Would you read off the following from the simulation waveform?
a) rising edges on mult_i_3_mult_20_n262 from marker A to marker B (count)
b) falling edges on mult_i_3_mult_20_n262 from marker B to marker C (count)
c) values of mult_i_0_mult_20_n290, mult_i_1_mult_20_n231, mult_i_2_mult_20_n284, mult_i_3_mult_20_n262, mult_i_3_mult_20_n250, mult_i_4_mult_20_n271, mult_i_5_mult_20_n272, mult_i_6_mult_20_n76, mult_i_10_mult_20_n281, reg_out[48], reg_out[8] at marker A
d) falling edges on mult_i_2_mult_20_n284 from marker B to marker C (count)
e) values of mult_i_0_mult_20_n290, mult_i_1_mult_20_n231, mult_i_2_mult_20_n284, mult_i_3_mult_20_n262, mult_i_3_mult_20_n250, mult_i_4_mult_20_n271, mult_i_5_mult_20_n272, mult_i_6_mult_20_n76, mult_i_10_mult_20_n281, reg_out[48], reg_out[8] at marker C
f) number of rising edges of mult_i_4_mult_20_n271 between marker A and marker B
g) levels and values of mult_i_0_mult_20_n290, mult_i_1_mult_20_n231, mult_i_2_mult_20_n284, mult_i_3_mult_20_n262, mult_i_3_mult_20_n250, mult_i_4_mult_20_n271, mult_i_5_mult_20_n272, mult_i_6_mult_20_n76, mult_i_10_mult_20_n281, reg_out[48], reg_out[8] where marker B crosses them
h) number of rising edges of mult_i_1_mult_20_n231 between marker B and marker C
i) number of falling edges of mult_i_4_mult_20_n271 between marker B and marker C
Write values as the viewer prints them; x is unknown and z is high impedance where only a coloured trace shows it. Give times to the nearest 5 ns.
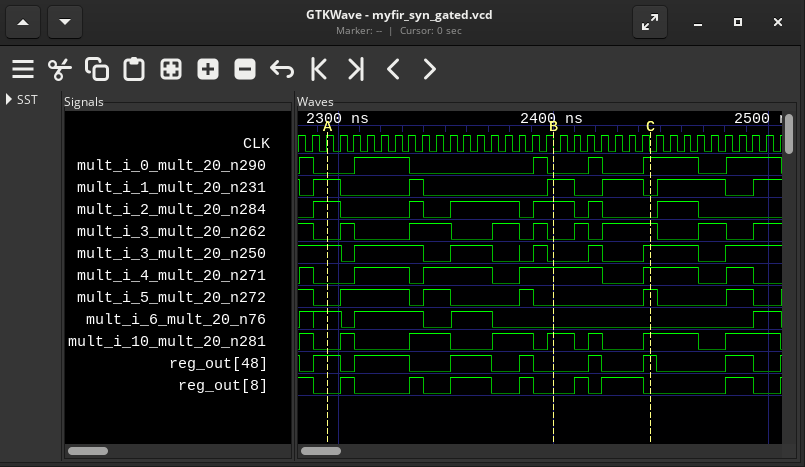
4
1
mult_i_0_mult_20_n290=0, mult_i_1_mult_20_n231=1, mult_i_2_mult_20_n284=1, mult_i_3_mult_20_n262=0, mult_i_3_mult_20_n250=1, mult_i_4_mult_20_n271=0, mult_i_5_mult_20_n272=0, mult_i_6_mult_20_n76=1, mult_i_10_mult_20_n281=0, reg_out[48]=1, reg_out[8]=0
2
mult_i_0_mult_20_n290=1, mult_i_1_mult_20_n231=0, mult_i_2_mult_20_n284=0, mult_i_3_mult_20_n262=1, mult_i_3_mult_20_n250=1, mult_i_4_mult_20_n271=1, mult_i_5_mult_20_n272=1, mult_i_6_mult_20_n76=0, mult_i_10_mult_20_n281=1, reg_out[48]=1, reg_out[8]=0
3
mult_i_0_mult_20_n290=0, mult_i_1_mult_20_n231=1, mult_i_2_mult_20_n284=1, mult_i_3_mult_20_n262=0, mult_i_3_mult_20_n250=0, mult_i_4_mult_20_n271=1, mult_i_5_mult_20_n272=0, mult_i_6_mult_20_n76=0, mult_i_10_mult_20_n281=1, reg_out[48]=0, reg_out[8]=0
1
1
